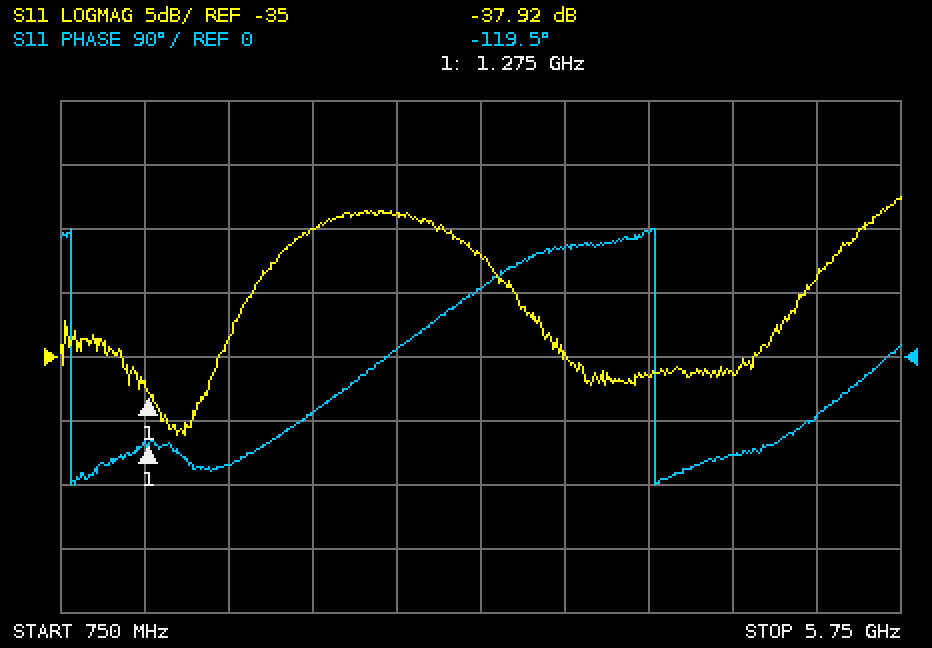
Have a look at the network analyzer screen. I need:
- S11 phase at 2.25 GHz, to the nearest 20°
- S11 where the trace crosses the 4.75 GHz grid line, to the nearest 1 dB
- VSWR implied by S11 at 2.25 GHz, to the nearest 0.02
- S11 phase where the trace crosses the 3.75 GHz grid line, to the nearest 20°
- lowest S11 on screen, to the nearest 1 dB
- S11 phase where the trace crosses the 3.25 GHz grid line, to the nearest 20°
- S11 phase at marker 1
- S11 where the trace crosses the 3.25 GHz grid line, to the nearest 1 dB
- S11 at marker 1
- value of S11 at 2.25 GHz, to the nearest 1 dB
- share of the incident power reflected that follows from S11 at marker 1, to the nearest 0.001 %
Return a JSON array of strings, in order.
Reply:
["-80°", "-36 dB", "1.12", "160°", "-41 dB", "100°", "-119.5°", "-27 dB", "-37.92 dB", "-25 dB", "0.016 %"]
